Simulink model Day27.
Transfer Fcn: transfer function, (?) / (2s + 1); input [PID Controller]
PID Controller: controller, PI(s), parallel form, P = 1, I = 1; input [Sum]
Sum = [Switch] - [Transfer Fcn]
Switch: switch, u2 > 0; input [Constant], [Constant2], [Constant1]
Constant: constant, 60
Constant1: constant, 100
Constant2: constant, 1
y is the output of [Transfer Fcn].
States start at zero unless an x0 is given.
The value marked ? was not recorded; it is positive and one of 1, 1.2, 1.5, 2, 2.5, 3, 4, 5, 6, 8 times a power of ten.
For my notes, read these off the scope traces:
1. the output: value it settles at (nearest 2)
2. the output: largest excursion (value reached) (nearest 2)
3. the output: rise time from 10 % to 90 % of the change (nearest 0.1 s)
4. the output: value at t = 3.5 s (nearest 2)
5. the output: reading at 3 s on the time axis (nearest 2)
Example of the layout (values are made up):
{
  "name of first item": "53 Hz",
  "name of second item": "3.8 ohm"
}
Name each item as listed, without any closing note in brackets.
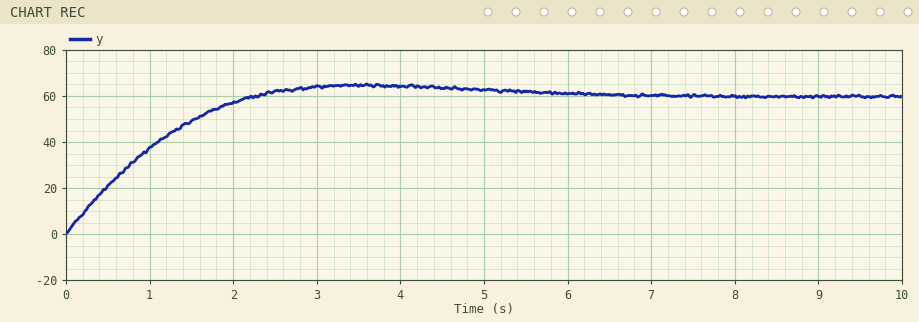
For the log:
{
  "the output: value it settles at": "60",
  "the output: largest excursion (value reached)": "64",
  "the output: rise time from 10 % to 90 % of the change": "1.6 s",
  "the output: value at t = 3.5 s": "64",
  "the output: reading at 3 s on the time axis": "64"
}
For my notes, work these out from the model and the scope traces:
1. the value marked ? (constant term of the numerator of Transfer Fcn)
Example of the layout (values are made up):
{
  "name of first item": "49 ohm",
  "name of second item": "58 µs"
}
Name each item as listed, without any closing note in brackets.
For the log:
{
  "the value marked ?": "1.5"
}
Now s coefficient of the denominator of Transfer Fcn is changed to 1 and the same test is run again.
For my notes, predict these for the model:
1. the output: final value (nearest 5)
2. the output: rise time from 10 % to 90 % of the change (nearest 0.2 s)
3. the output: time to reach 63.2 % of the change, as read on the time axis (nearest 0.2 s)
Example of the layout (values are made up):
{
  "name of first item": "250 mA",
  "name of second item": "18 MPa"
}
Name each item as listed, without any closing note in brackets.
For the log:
{
  "the output: final value": "60",
  "the output: rise time from 10 % to 90 % of the change": "1.4 s",
  "the output: time to reach 63.2 % of the change, as read on the time axis": "0.6 s"
}
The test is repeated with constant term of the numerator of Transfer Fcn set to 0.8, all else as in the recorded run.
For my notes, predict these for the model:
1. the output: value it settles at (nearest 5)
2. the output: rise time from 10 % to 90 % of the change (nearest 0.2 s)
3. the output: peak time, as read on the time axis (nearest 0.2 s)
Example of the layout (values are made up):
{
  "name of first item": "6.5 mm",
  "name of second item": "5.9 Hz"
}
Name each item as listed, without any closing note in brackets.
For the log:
{
  "the output: value it settles at": "60",
  "the output: rise time from 10 % to 90 % of the change": "2.6 s",
  "the output: peak time, as read on the time axis": "5.6 s"
}
